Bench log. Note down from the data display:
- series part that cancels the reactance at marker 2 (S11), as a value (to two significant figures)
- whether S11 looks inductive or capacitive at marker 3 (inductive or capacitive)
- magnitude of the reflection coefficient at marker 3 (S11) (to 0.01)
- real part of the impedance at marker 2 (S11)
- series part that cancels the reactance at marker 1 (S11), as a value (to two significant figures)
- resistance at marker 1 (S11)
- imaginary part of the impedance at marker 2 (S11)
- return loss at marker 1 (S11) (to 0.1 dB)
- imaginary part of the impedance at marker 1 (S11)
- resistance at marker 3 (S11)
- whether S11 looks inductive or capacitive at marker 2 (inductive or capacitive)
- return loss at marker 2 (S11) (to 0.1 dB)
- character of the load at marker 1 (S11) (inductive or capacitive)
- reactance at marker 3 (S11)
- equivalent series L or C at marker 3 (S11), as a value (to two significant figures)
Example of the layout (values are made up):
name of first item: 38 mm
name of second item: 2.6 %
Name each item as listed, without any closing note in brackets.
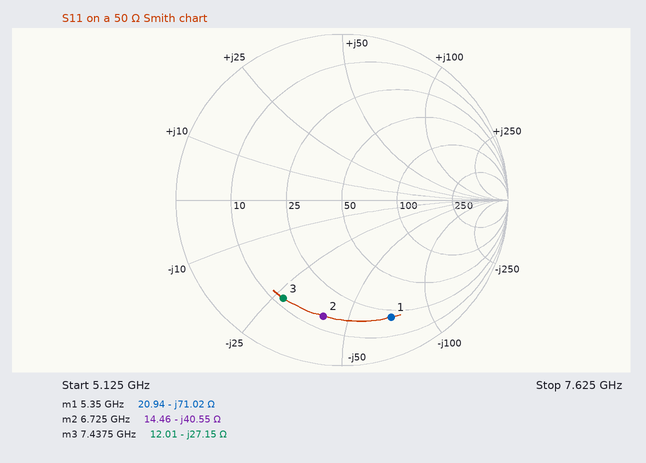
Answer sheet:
series part that cancels the reactance at marker 2 (S11), as a value: 960 pH
whether S11 looks inductive or capacitive at marker 3: capacitive
magnitude of the reflection coefficient at marker 3 (S11): 0.69
real part of the impedance at marker 2: 14.46 Ω
series part that cancels the reactance at marker 1 (S11), as a value: 2.1 nH
resistance at marker 1: 20.94 Ω
imaginary part of the impedance at marker 2: -40.55 Ω
return loss at marker 1 (S11): 2.3 dB
imaginary part of the impedance at marker 1: -71.02 Ω
resistance at marker 3: 12.01 Ω
whether S11 looks inductive or capacitive at marker 2: capacitive
return loss at marker 2 (S11): 3.0 dB
character of the load at marker 1 (S11): capacitive
reactance at marker 3: -27.15 Ω
equivalent series L or C at marker 3 (S11), as a value: 790 fF
